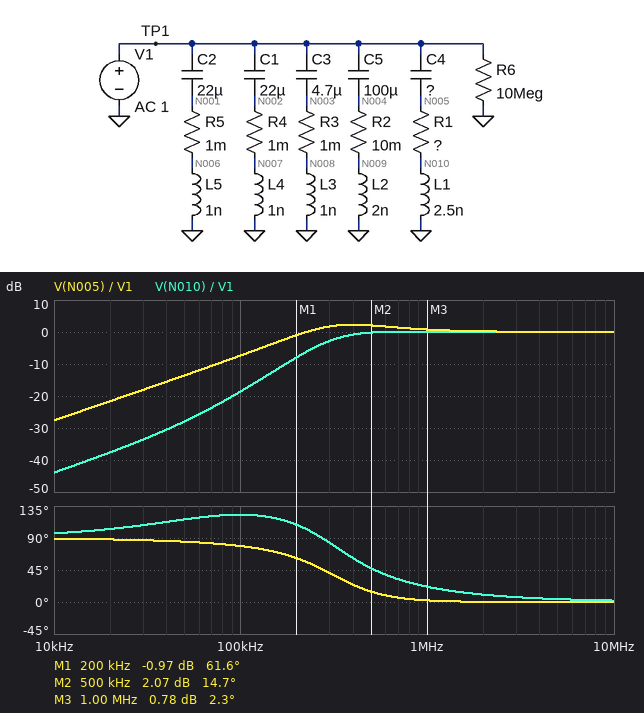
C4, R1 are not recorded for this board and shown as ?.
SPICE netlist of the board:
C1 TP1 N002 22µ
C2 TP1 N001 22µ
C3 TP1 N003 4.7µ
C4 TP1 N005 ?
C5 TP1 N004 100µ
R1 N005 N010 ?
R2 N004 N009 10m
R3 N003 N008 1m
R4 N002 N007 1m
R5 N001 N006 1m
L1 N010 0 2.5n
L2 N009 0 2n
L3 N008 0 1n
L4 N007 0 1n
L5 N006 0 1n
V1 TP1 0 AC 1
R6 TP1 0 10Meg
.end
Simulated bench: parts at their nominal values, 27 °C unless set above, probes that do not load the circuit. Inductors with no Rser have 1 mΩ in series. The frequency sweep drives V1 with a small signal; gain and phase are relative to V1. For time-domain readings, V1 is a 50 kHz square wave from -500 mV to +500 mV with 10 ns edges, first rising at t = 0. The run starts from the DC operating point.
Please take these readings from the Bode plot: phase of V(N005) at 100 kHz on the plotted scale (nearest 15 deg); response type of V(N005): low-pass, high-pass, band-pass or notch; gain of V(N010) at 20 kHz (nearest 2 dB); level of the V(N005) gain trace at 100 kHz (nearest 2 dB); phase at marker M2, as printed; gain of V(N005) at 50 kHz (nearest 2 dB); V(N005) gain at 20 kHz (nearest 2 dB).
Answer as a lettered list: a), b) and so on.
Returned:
a) 75 deg
b) high-pass
c) -38 dB
d) -8 dB
e) 14.7 deg
f) -14 dB
g) -22 dB
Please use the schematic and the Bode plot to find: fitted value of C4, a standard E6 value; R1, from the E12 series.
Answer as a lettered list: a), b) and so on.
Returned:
a) 100 µF
b) 5.6 mΩ
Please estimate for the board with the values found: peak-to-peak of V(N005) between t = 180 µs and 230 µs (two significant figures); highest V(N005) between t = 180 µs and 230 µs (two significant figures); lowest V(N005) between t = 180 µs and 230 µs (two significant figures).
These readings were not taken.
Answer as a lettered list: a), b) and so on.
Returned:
a) 2.0 V
b) 1.0 V
c) -1.0 V
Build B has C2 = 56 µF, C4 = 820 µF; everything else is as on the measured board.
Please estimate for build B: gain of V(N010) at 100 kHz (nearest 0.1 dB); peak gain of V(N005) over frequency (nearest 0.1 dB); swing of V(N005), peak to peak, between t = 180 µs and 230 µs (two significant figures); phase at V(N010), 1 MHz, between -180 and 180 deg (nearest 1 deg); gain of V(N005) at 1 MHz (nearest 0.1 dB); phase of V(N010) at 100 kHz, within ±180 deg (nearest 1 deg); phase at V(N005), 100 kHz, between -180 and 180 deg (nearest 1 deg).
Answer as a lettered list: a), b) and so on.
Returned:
a) -11.0 dB
b) 0.4 dB
c) 1.7 V
d) 19 deg
e) 0.1 dB
f) 61 deg
g) 17 deg
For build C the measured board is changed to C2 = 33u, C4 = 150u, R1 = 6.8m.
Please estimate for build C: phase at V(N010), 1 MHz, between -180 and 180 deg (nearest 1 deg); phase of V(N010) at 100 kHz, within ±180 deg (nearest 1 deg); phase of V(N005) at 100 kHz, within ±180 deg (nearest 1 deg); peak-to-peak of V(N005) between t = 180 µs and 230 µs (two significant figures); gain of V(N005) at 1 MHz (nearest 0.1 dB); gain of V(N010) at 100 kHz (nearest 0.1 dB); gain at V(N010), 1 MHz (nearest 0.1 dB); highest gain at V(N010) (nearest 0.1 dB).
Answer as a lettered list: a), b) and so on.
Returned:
a) 24 deg
b) 107 deg
c) 61 deg
d) 2.0 V
e) 0.5 dB
f) -16.1 dB
g) -0.5 dB
h) 0 dB
